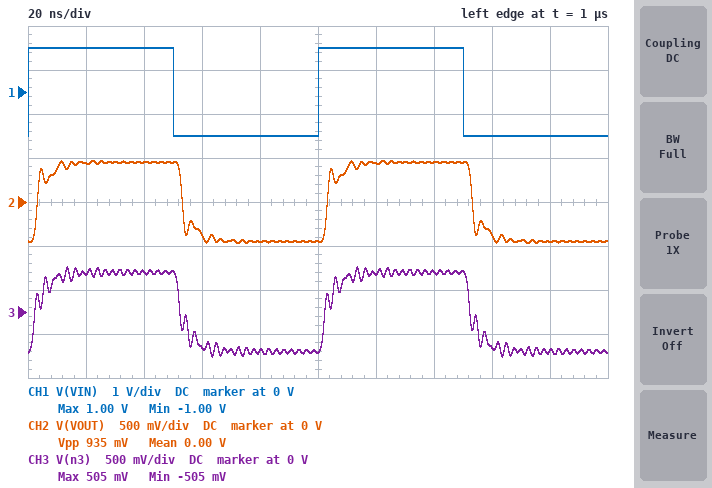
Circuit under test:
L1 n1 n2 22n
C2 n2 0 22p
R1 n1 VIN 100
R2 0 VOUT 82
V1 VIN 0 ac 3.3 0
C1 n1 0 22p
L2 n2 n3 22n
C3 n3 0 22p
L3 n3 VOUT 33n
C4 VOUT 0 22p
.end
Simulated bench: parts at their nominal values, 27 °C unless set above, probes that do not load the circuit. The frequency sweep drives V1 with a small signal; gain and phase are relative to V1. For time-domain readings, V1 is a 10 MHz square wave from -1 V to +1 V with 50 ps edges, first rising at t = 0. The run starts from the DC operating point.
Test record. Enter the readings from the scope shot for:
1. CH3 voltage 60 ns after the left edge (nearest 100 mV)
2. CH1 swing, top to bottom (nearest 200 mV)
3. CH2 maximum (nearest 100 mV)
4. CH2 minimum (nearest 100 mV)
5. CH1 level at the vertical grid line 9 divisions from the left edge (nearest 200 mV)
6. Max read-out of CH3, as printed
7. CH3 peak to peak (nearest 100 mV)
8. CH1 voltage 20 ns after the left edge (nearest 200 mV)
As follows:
-400 mV
2.0 V
500 mV
-500 mV
-1.0 V
505 mV
1.0 V
1.0 V
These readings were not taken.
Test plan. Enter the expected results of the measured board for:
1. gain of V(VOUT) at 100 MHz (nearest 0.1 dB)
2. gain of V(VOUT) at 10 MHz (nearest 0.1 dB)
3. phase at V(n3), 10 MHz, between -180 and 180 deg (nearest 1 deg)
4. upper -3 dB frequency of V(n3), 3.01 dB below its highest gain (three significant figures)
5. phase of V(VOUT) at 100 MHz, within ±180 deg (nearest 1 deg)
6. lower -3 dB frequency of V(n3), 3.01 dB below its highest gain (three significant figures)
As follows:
-10.4 dB
-7.1 dB
-14 deg
412 MHz
-94 deg
402 MHz
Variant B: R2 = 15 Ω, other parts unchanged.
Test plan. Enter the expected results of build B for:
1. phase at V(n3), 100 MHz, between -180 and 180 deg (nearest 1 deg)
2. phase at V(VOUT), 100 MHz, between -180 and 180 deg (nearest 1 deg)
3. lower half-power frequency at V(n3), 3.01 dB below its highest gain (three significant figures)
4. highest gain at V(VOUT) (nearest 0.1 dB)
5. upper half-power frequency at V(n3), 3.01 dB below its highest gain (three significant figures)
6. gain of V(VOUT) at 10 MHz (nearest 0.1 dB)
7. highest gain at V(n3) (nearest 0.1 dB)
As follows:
-41 deg
-104 deg
399 MHz
-14.4 dB
411 MHz
-17.6 dB
1.2 dB
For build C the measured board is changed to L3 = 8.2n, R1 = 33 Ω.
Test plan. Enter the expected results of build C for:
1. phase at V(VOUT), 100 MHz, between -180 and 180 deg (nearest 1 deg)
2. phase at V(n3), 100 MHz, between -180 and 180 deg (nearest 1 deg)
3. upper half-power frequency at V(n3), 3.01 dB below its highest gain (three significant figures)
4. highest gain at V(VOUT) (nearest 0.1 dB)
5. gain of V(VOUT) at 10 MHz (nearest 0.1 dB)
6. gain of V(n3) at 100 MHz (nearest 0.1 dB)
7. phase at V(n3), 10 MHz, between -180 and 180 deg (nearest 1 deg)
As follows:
-82 deg
-78 deg
176 MHz
-2.9 dB
-3.0 dB
-4.3 dB
-9 deg
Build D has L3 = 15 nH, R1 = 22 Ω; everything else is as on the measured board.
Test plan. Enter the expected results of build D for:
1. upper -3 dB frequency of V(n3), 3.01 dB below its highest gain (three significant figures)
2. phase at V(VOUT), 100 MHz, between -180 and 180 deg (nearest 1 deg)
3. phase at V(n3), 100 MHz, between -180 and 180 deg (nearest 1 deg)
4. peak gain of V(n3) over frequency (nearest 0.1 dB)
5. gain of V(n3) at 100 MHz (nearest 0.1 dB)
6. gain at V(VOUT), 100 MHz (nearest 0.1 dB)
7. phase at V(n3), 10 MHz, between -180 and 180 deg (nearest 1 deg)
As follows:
460 MHz
-85 deg
-77 deg
2.3 dB
-2.0 dB
-0.9 dB
-7 deg
